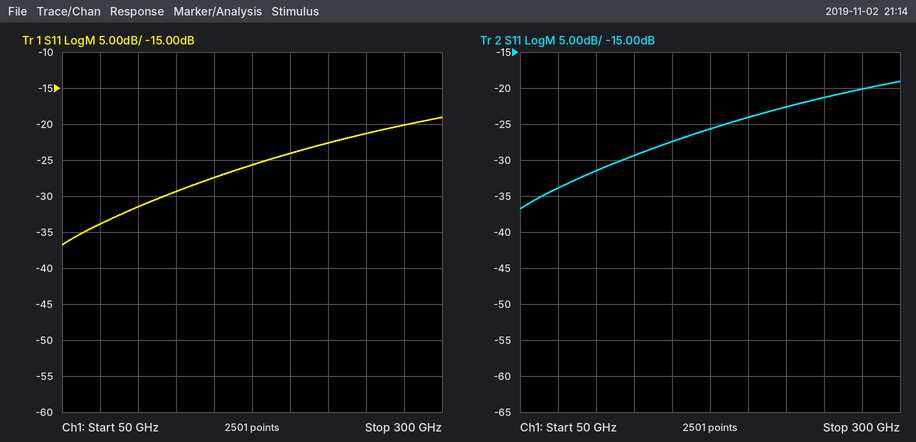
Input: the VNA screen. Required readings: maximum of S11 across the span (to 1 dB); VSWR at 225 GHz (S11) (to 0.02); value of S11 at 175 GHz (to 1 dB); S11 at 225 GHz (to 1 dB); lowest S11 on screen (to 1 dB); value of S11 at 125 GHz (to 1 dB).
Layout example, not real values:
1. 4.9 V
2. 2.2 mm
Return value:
1. -19 dB
2. 1.16
3. -26 dB
4. -23 dB
5. -37 dB
6. -29 dB
